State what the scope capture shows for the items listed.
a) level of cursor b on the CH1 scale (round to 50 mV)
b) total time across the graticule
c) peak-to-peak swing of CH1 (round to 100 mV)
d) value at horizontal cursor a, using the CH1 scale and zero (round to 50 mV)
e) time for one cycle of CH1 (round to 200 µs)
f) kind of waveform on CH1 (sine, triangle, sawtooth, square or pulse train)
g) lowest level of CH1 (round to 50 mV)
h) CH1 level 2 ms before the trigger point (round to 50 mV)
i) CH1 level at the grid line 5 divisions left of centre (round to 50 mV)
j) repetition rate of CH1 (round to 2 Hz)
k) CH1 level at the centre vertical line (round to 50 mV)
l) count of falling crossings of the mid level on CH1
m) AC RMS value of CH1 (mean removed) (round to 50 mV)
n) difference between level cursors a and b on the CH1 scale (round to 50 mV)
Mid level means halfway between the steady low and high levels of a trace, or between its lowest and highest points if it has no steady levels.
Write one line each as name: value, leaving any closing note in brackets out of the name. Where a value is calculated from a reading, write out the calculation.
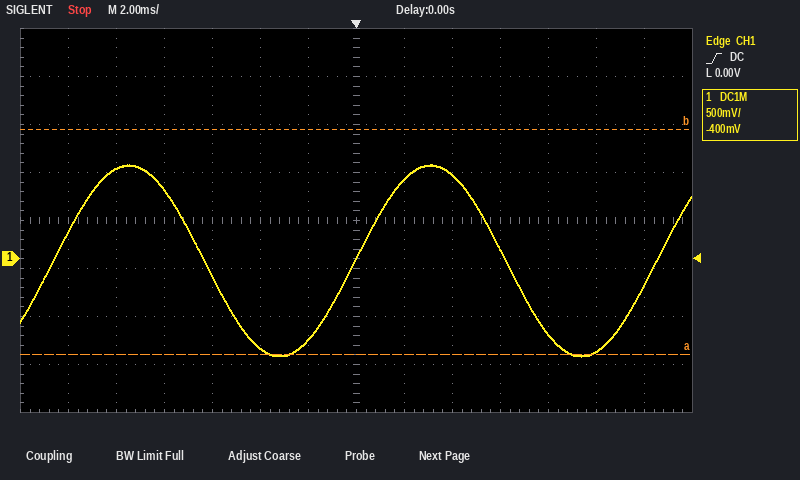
level of cursor b on the CH1 scale: 1.35 V
total time across the graticule: 28 ms
peak-to-peak swing of CH1: 2.00 V
value at horizontal cursor a, using the CH1 scale and zero: -1.00 V
time for one cycle of CH1: 12.6 ms
kind of waveform on CH1: sine
lowest level of CH1: -1.00 V
CH1 level 2 ms before the trigger point: -850 mV
CH1 level at the grid line 5 divisions left of centre: 950 mV
repetition rate of CH1: 1 / 12.6 ms ≈ 79.4 Hz, so 80 Hz to the nearest 2 Hz
CH1 level at the centre vertical line: 0 mV
count of falling crossings of the mid level on CH1: 2
AC RMS value of CH1 (mean removed): 2.00 V / (2√2) ≈ 707 mV, so 700 mV to the nearest 50 mV
difference between level cursors a and b on the CH1 scale: 2.35 V
